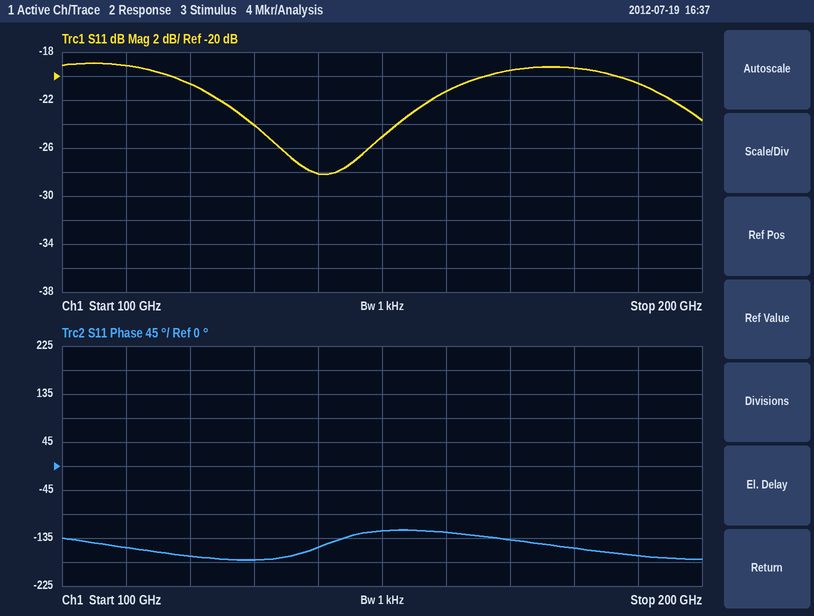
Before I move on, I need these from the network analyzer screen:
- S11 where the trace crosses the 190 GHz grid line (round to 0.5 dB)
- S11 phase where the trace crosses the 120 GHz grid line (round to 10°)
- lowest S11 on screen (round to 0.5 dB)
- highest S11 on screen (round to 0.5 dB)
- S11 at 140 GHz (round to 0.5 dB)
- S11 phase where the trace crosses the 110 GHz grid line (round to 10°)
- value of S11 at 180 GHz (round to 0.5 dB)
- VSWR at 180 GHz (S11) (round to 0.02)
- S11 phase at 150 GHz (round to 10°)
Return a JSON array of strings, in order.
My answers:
["-20.5 dB", "-170°", "-28.0 dB", "-19.0 dB", "-28.0 dB", "-150°", "-19.5 dB", "1.24", "-120°"]
